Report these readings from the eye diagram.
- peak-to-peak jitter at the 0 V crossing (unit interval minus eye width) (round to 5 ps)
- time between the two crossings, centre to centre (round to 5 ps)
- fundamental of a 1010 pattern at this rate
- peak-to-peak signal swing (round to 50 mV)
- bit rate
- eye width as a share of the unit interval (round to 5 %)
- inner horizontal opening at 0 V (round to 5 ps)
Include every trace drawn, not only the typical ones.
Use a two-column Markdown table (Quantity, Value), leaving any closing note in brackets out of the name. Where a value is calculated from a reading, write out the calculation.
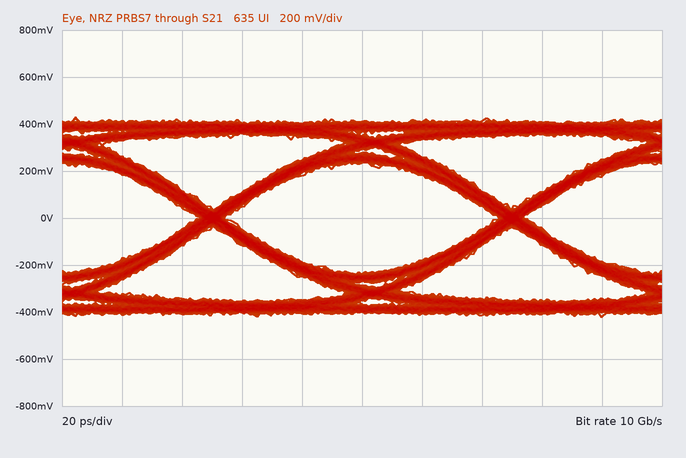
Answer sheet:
| Quantity | Value |
|---|---|
| peak-to-peak jitter at the 0 V crossing (unit interval minus eye width) | 10 ps |
| time between the two crossings, centre to centre | 100 ps |
| fundamental of a 1010 pattern at this rate | 5 GHz |
| peak-to-peak signal swing | 850 mV |
| bit rate | 10 Gb/s |
| eye width as a share of the unit interval | 90 ps / 100 ps ≈ 90 % |
| inner horizontal opening at 0 V | 90 ps |
